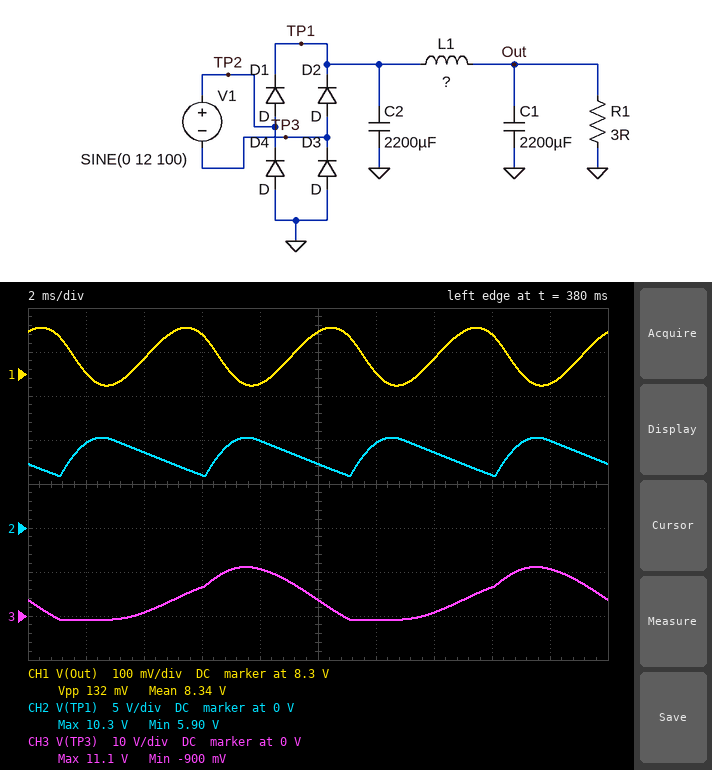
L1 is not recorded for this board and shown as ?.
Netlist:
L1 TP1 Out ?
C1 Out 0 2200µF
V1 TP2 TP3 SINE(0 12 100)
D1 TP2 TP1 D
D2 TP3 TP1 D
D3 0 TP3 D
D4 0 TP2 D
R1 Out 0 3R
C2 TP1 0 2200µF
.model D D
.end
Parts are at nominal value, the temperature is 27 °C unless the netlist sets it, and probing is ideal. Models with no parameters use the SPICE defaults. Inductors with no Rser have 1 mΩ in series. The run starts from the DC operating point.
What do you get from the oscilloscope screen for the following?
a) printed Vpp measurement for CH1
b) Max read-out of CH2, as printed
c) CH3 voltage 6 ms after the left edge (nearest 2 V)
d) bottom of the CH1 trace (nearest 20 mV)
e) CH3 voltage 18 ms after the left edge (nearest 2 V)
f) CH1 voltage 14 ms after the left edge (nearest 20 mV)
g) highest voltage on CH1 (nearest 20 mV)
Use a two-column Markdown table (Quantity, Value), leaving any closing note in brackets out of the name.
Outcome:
| Quantity | Value |
|---|---|
| printed Vpp measurement for CH1 | 132 mV |
| Max read-out of CH2, as printed | 10.3 V |
| CH3 voltage 6 ms after the left edge | 6 V |
| bottom of the CH1 trace | 8.28 V |
| CH3 voltage 18 ms after the left edge | 10 V |
| CH1 voltage 14 ms after the left edge | 8.34 V |
| highest voltage on CH1 | 8.40 V |
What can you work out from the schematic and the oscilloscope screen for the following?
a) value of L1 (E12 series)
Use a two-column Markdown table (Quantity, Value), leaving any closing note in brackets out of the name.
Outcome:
| Quantity | Value |
|---|---|
| value of L1 | 8.2 mH |
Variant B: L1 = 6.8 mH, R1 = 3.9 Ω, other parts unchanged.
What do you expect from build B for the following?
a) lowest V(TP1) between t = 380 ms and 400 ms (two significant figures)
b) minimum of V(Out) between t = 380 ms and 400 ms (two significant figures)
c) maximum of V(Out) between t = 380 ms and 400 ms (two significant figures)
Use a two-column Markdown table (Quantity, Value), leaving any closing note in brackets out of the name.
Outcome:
| Quantity | Value |
|---|---|
| lowest V(TP1) between t = 380 ms and 400 ms | 6.6 V |
| minimum of V(Out) between t = 380 ms and 400 ms | 8.6 V |
| maximum of V(Out) between t = 380 ms and 400 ms | 8.7 V |
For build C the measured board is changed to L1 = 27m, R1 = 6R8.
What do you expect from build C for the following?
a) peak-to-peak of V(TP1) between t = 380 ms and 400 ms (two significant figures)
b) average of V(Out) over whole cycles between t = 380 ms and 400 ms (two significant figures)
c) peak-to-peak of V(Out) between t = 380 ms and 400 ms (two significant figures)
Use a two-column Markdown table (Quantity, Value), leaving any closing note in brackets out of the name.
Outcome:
| Quantity | Value |
|---|---|
| peak-to-peak of V(TP1) between t = 380 ms and 400 ms | 2.4 V |
| average of V(Out) over whole cycles between t = 380 ms and 400 ms | 9.2 V |
| peak-to-peak of V(Out) between t = 380 ms and 400 ms | 20 mV |
